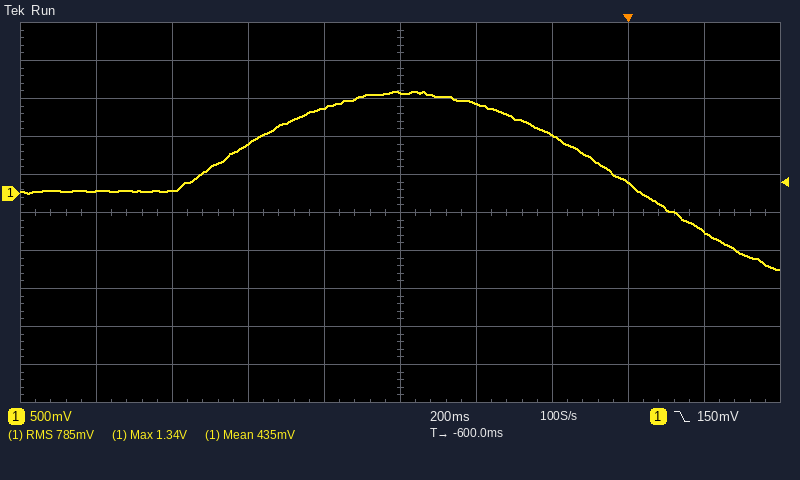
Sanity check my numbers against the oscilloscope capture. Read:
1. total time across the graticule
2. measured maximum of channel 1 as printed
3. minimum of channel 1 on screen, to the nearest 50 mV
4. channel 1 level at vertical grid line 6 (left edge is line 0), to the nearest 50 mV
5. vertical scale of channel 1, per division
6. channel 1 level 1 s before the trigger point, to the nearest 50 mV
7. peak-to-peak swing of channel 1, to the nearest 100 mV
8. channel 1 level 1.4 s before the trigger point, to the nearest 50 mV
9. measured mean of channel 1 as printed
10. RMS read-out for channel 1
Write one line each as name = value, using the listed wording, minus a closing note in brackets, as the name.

total time across the graticule = 2 s
measured maximum of channel 1 as printed = 1.34 V
minimum of channel 1 on screen, to the nearest 50 mV = -1.00 V
channel 1 level at vertical grid line 6 (left edge is line 0), to the nearest 50 mV = 1.20 V
vertical scale of channel 1, per division = 500 mV
channel 1 level 1 s before the trigger point, to the nearest 50 mV = 650 mV
peak-to-peak swing of channel 1, to the nearest 100 mV = 2.30 V
channel 1 level 1.4 s before the trigger point, to the nearest 50 mV = 50 mV
measured mean of channel 1 as printed = 435 mV
RMS read-out for channel 1 = 785 mV
